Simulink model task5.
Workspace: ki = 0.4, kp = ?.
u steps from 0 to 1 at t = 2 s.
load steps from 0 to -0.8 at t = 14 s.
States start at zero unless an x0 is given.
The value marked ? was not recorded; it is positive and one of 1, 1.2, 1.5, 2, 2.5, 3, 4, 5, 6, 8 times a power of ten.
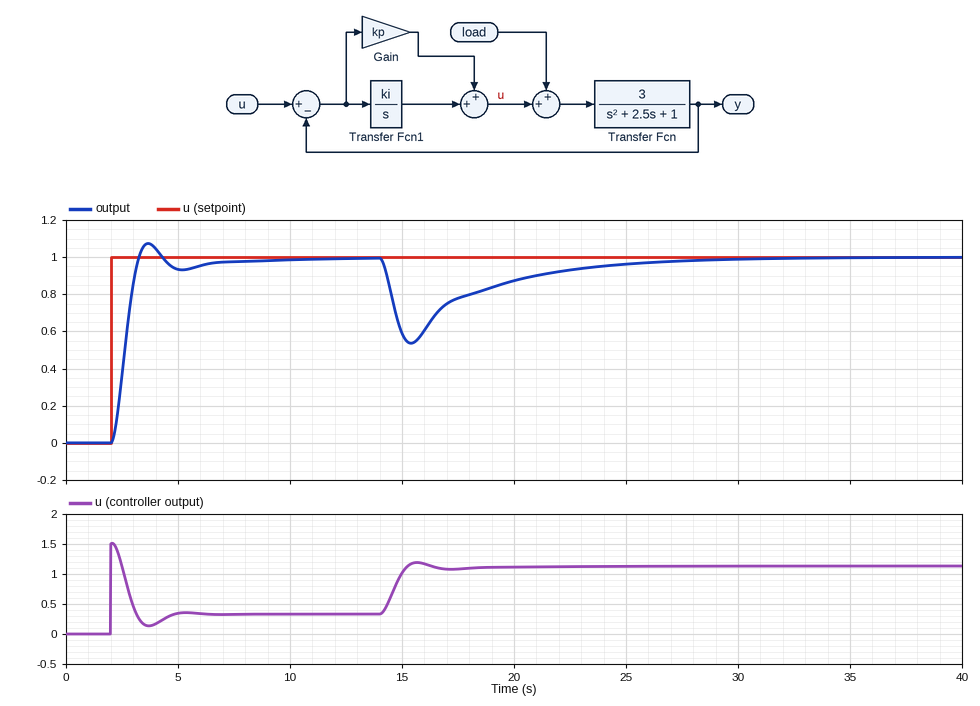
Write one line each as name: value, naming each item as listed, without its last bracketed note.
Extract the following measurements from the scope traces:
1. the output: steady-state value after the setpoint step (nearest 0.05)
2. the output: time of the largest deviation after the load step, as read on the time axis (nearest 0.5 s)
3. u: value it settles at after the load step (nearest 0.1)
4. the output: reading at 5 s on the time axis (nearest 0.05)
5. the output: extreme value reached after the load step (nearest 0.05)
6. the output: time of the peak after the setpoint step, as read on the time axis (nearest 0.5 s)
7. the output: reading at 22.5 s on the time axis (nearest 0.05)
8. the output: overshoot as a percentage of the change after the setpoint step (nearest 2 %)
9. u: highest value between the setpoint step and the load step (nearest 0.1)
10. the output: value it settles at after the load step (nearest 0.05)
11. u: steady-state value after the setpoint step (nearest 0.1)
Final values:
the output: steady-state value after the setpoint step: 1.00
the output: time of the largest deviation after the load step, as read on the time axis: 15.5 s
u: value it settles at after the load step: 1.1
the output: reading at 5 s on the time axis: 0.95
the output: extreme value reached after the load step: 0.55
the output: time of the peak after the setpoint step, as read on the time axis: 3.5 s
the output: reading at 22.5 s on the time axis: 0.95
the output: overshoot as a percentage of the change after the setpoint step: 8 %
u: highest value between the setpoint step and the load step: 1.5
the output: value it settles at after the load step: 1.00
u: steady-state value after the setpoint step: 0.3
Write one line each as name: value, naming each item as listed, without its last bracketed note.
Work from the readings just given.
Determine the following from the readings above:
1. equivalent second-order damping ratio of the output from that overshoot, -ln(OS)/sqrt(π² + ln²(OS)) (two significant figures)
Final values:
equivalent second-order damping ratio of the output from that overshoot, -ln(OS)/sqrt(π² + ln²(OS)): 0.63
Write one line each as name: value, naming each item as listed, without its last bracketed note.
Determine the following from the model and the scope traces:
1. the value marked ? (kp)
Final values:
the value marked ?: 1.5
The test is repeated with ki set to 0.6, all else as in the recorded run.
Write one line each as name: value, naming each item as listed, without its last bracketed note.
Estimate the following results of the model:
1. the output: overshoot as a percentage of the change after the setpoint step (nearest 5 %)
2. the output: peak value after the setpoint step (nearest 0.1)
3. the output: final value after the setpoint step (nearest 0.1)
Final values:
the output: overshoot as a percentage of the change after the setpoint step: 15 %
the output: peak value after the setpoint step: 1.1
the output: final value after the setpoint step: 1.0
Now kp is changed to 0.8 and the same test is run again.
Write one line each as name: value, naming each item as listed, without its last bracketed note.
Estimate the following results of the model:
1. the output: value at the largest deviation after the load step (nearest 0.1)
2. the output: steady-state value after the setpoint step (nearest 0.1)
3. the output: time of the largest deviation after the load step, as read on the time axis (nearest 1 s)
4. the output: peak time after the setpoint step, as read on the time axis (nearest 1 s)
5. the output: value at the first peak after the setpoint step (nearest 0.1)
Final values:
the output: value at the largest deviation after the load step: 0.4
the output: steady-state value after the setpoint step: 1.0
the output: time of the largest deviation after the load step, as read on the time axis: 16 s
the output: peak time after the setpoint step, as read on the time axis: 5 s
the output: value at the first peak after the setpoint step: 1.1
